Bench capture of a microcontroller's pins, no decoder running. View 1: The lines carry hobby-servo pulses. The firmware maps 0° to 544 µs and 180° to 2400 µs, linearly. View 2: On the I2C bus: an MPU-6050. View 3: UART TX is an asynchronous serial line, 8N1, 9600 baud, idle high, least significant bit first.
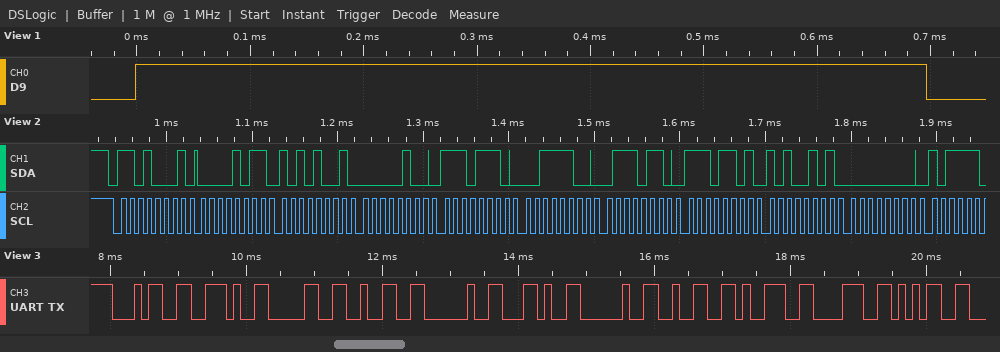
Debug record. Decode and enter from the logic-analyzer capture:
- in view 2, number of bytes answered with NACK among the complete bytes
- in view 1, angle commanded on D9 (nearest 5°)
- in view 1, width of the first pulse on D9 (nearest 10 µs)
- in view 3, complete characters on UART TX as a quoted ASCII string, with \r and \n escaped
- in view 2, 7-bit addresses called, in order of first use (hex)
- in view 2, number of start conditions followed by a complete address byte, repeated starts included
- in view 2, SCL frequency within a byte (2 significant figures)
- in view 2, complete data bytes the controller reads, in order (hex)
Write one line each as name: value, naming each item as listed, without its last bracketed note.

in view 2, number of bytes answered with NACK among the complete bytes: 0
in view 1, angle commanded on D9: 15°
in view 1, width of the first pulse on D9: 700 µs
in view 3, complete characters on UART TX as a quoted ASCII string, with \r and \n escaped: "4.02 , 2985"
in view 2, 7-bit addresses called, in order of first use: 0x68
in view 2, number of start conditions followed by a complete address byte, repeated starts included: 1
in view 2, SCL frequency within a byte: 100 kHz
in view 2, complete data bytes the controller reads, in order: 0B A9 04 EE 3C 76 ED A5 00
